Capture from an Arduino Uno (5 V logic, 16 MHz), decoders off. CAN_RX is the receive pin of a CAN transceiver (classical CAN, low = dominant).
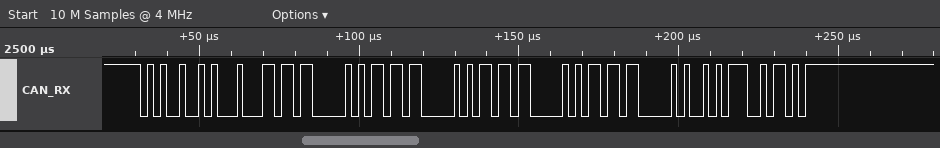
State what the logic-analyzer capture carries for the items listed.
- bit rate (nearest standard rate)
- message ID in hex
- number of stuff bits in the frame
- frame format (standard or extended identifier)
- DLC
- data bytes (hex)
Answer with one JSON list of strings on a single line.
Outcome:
["500 kbit/s", "0x525", "4", "standard", "8", "DB 02 DB 02 DB 02 DB 02"]
